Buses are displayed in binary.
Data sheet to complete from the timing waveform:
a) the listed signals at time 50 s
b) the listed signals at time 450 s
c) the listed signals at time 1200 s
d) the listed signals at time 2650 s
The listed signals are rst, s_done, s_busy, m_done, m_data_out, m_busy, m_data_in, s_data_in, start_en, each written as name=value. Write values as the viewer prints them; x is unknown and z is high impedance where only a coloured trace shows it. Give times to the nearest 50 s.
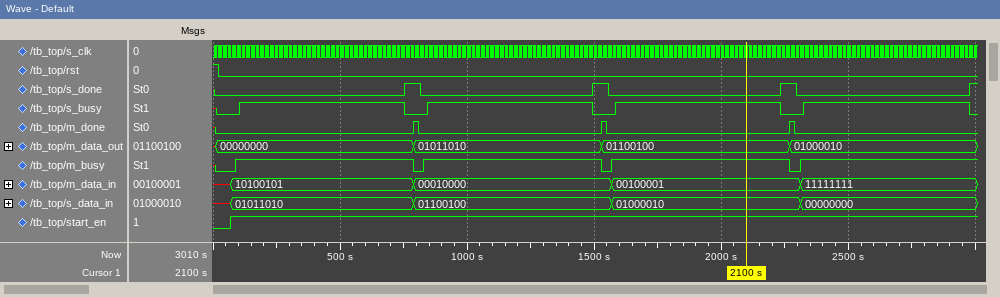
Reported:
rst=0, s_done=0, s_busy=0, m_done=0, m_data_out=00000000, m_busy=0, m_data_in=x, s_data_in=x, start_en=0
rst=0, s_done=0, s_busy=1, m_done=0, m_data_out=00000000, m_busy=1, m_data_in=10100101, s_data_in=01011010, start_en=1
rst=0, s_done=0, s_busy=1, m_done=0, m_data_out=01011010, m_busy=1, m_data_in=00010000, s_data_in=01100100, start_en=1
rst=0, s_done=0, s_busy=1, m_done=0, m_data_out=01000010, m_busy=1, m_data_in=11111111, s_data_in=00000000, start_en=1
